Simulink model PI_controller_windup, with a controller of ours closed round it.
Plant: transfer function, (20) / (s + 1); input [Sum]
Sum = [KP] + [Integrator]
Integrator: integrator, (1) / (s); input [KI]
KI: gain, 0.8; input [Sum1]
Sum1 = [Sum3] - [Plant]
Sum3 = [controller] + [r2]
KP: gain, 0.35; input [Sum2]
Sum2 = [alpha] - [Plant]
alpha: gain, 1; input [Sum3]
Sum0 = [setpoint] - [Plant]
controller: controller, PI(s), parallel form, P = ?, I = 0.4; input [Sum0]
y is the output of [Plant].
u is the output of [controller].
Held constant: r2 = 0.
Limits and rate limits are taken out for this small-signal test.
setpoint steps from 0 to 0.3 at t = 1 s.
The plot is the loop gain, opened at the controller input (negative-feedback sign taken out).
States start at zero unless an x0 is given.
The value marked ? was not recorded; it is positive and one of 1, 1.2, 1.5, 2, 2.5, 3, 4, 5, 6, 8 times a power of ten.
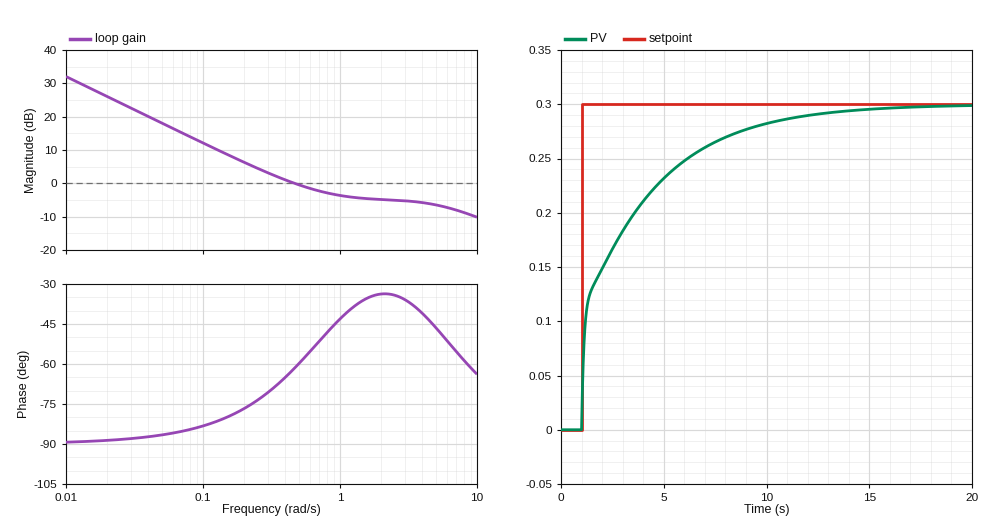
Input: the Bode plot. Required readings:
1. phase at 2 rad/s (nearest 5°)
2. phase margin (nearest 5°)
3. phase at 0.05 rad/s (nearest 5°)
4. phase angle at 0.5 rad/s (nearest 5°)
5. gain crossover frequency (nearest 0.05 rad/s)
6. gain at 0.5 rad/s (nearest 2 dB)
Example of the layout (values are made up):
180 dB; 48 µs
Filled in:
-35°; 120°; -85°; -60°; 0.45 rad/s; 0 dB
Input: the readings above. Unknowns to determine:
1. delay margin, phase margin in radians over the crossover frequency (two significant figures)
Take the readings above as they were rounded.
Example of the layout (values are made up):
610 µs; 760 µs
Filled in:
4.7 s
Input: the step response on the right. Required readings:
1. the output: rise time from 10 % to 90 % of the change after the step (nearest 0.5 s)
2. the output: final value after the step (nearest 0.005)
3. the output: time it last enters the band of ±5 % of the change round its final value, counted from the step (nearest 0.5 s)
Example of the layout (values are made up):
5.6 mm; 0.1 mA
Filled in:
7.0 s; 0.300; 9.5 s
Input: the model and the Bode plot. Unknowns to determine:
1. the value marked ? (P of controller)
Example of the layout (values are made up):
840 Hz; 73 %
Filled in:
0.5
